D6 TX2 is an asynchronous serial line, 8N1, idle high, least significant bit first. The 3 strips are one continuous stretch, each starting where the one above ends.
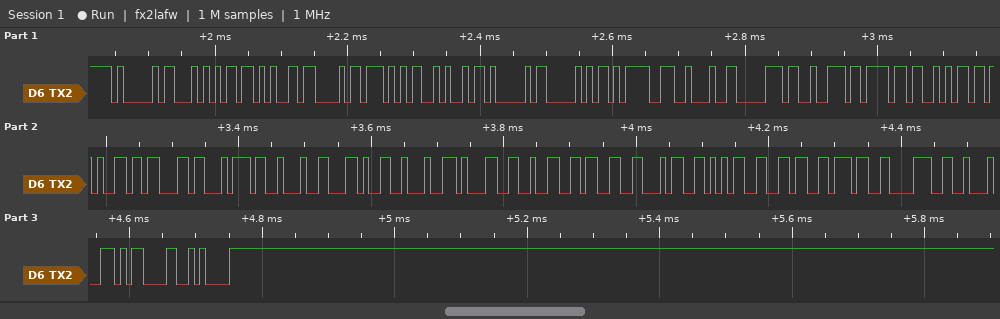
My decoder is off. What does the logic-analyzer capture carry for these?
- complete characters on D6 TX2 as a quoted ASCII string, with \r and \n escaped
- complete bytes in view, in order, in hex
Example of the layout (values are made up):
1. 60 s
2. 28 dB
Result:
1. "AT+CWJAP=\"project\",\"12345678\"\r\n"
2. 41 54 2B 43 57 4A 41 50 3D 22 70 72 6F 6A 65 63 74 22 2C 22 31 32 33 34 35 36 37 38 22 0D 0A
